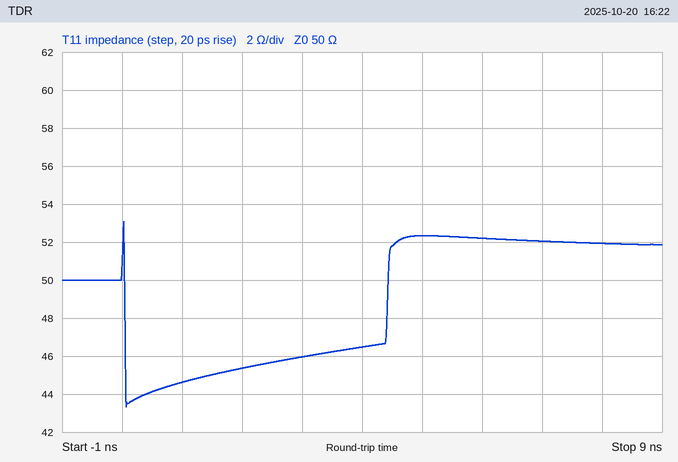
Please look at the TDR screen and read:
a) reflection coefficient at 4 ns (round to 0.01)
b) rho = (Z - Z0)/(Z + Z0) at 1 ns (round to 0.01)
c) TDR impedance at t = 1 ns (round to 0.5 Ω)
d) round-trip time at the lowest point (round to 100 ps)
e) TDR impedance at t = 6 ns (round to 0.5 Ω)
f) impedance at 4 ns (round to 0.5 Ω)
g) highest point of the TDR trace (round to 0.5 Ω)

-0.04
-0.06
44.5 Ω
100 ps
52.0 Ω
46.5 Ω
53.0 Ω
